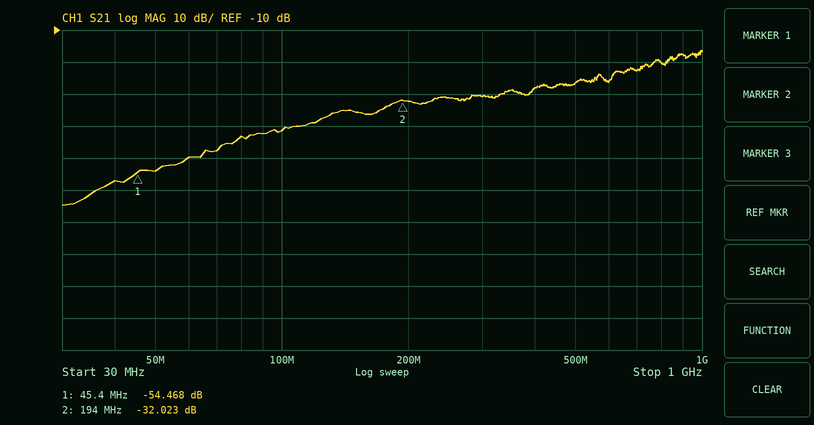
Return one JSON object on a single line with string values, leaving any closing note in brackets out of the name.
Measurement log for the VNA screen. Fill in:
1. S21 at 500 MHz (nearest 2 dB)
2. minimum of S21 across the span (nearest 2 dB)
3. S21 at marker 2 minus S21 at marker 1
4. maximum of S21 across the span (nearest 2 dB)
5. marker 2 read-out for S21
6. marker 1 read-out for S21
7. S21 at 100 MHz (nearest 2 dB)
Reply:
{"S21 at 500 MHz": "-26 dB", "minimum of S21 across the span": "-64 dB", "S21 at marker 2 minus S21 at marker 1": "22.445 dB", "maximum of S21 across the span": "-16 dB", "marker 2 read-out for S21": "-32.023 dB", "marker 1 read-out for S21": "-54.468 dB", "S21 at 100 MHz": "-42 dB"}
